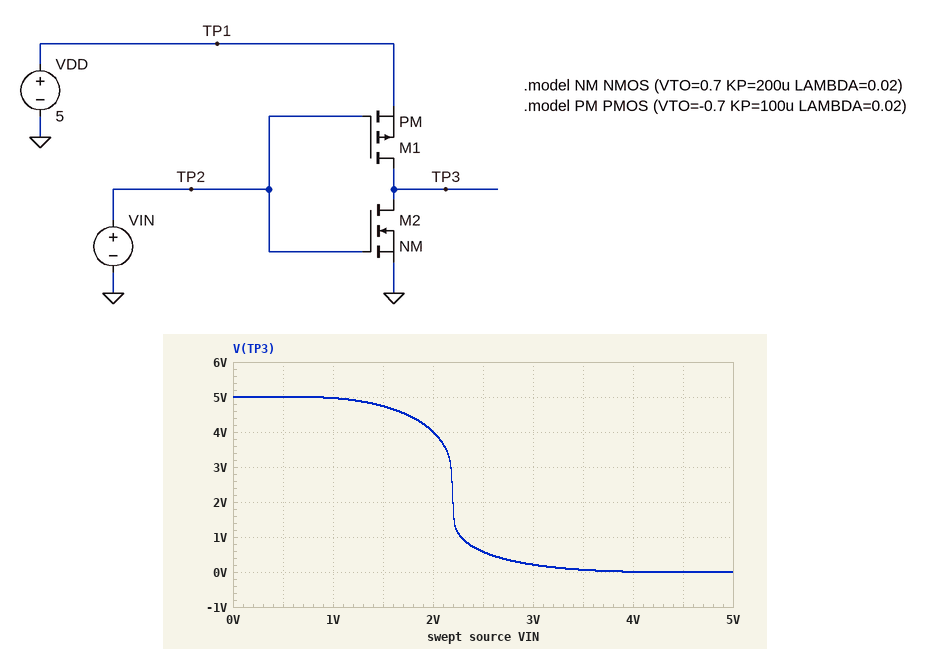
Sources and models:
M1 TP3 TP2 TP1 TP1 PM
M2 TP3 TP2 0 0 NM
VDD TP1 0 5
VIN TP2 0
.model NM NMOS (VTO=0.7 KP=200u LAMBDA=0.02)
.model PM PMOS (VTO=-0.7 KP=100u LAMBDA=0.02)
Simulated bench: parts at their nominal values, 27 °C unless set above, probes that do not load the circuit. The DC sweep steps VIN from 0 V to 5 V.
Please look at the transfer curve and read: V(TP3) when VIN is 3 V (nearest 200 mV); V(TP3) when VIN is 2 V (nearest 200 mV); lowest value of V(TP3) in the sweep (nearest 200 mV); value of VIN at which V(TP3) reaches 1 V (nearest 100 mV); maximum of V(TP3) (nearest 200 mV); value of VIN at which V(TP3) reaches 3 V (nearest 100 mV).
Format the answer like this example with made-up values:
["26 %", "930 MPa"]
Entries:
["200 mV", "4.0 V", "0 V", "2.3 V", "5.0 V", "2.2 V"]
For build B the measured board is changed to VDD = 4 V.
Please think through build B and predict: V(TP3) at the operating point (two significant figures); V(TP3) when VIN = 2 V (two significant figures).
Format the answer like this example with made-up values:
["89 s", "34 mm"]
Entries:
["4.0 V", "410 mV"]
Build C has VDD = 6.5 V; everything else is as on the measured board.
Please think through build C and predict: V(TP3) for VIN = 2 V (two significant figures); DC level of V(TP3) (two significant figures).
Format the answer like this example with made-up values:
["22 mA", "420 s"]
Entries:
["6.0 V", "6.5 V"]
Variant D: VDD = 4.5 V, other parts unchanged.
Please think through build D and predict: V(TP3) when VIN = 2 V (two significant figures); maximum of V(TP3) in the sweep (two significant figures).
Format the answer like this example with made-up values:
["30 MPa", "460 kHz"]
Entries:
["1.2 V", "4.5 V"]
